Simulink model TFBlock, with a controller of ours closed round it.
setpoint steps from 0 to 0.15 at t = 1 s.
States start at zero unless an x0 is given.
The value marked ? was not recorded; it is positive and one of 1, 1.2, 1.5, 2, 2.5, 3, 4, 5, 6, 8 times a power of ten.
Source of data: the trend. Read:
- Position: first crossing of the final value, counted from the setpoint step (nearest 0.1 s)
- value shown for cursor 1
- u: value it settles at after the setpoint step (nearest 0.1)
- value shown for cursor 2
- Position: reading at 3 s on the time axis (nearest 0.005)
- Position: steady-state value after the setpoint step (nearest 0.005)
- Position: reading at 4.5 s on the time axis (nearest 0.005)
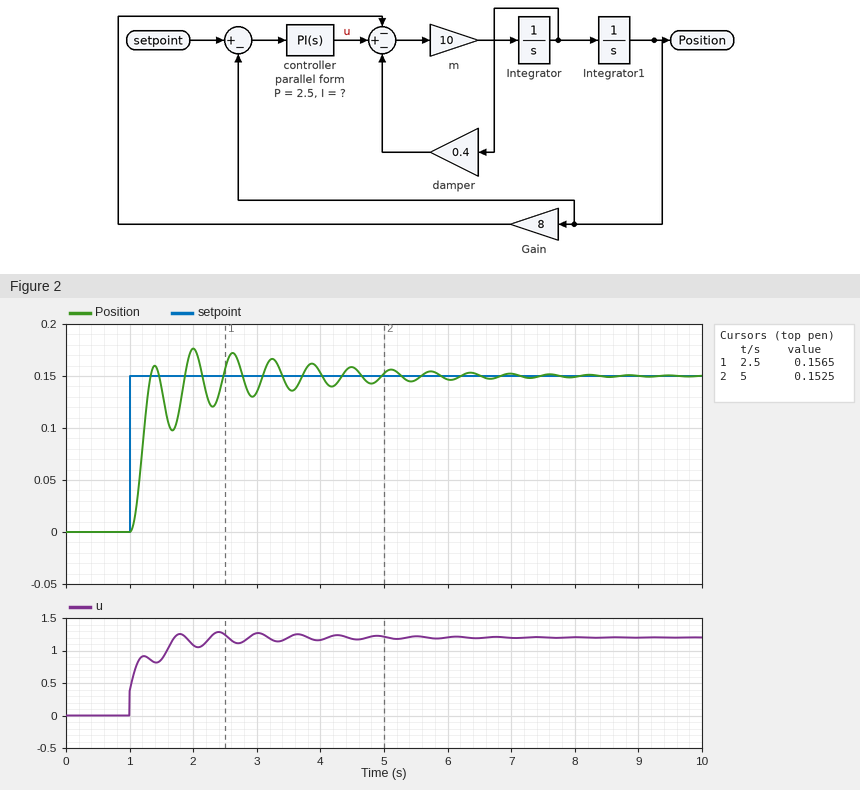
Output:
0.3 s
0.1565
1.2
0.1525
0.135
0.150
0.160
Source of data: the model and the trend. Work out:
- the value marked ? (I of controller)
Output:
30
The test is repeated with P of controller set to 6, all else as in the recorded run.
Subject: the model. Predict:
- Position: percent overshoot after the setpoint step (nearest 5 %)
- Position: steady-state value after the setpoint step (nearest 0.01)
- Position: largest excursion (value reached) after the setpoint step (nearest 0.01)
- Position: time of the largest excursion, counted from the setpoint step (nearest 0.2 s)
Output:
15 %
0.15
0.17
0.8 s
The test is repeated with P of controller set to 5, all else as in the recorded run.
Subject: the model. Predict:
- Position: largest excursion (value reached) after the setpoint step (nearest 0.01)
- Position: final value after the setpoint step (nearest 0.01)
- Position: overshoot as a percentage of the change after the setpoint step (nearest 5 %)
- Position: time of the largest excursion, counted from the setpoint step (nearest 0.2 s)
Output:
0.17
0.15
15 %
0.8 s
